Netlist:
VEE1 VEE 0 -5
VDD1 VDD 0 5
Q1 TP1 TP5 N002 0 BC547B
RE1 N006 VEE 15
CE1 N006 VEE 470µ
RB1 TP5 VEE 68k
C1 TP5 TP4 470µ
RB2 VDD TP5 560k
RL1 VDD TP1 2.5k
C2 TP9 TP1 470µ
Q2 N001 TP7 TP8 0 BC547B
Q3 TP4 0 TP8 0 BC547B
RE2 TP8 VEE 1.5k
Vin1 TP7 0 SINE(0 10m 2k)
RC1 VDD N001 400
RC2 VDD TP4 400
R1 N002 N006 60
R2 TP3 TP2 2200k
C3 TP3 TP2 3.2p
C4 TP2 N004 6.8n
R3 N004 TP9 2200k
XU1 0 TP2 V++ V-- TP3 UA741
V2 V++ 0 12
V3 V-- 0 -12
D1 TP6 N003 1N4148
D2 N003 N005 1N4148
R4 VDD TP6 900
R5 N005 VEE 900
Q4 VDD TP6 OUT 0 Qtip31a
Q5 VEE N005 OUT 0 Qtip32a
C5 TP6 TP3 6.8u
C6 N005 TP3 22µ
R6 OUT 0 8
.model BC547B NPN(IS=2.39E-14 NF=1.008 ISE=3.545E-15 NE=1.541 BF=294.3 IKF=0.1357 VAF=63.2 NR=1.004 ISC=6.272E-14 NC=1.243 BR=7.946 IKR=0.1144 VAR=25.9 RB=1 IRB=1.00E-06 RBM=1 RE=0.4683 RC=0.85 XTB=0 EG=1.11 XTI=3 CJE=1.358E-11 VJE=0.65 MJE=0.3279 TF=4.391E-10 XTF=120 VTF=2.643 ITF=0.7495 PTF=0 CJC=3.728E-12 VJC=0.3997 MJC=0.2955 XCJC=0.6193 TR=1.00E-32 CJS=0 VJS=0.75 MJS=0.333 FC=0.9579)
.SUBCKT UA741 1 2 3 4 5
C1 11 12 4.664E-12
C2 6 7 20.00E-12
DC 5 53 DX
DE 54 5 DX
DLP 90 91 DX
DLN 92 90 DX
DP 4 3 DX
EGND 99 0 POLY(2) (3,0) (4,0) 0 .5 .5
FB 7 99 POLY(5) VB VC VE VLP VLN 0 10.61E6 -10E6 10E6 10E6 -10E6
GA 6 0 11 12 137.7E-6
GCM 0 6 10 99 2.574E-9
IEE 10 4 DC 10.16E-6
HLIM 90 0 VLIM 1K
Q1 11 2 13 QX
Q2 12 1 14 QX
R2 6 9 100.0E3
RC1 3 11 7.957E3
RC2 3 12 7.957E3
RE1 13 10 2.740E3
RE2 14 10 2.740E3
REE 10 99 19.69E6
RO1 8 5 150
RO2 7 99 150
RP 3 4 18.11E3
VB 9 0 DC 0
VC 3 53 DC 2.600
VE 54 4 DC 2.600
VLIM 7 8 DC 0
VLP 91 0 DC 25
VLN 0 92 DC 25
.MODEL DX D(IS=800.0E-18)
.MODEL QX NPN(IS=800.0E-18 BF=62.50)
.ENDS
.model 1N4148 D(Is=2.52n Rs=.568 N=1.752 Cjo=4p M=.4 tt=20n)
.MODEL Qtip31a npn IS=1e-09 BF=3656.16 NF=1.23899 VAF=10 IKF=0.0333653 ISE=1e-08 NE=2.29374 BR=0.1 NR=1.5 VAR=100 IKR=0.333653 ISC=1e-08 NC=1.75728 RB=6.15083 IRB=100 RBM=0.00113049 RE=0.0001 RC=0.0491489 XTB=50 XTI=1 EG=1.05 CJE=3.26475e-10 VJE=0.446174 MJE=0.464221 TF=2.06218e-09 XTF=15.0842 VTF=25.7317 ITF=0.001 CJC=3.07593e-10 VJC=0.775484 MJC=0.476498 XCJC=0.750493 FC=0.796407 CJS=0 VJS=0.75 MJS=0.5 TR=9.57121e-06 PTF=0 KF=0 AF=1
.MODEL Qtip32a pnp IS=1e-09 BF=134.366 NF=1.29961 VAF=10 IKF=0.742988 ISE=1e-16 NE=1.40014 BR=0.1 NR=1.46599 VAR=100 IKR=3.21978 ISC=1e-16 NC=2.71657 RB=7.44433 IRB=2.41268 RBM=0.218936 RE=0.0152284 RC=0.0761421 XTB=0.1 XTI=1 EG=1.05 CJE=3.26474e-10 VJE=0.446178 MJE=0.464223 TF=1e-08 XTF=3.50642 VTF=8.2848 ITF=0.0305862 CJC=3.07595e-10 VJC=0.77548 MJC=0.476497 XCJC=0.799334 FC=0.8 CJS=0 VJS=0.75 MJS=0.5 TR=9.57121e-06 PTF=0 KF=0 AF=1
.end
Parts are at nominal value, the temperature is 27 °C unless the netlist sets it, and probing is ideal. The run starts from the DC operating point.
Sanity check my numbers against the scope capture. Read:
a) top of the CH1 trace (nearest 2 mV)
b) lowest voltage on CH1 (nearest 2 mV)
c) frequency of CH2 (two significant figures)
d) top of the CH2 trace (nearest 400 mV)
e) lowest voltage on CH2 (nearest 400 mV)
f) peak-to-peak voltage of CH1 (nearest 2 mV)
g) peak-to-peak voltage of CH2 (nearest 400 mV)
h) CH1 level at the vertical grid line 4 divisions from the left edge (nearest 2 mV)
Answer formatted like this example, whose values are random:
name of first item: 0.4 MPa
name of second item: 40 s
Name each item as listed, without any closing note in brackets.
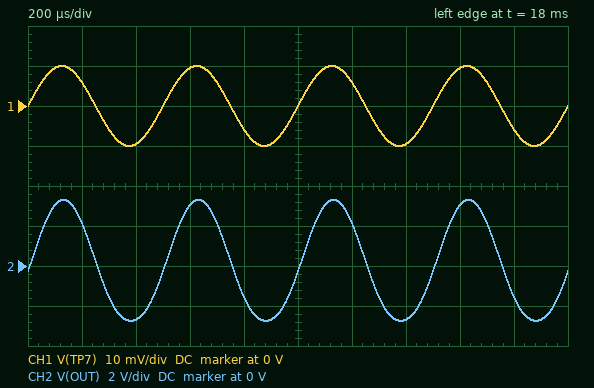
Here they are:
top of the CH1 trace: 10 mV
lowest voltage on CH1: -10 mV
frequency of CH2: 2.0 kHz
top of the CH2 trace: 3.2 V
lowest voltage on CH2: -2.8 V
peak-to-peak voltage of CH1: 20 mV
peak-to-peak voltage of CH2: 6.0 V
CH1 level at the vertical grid line 4 divisions from the left edge: -6 mV
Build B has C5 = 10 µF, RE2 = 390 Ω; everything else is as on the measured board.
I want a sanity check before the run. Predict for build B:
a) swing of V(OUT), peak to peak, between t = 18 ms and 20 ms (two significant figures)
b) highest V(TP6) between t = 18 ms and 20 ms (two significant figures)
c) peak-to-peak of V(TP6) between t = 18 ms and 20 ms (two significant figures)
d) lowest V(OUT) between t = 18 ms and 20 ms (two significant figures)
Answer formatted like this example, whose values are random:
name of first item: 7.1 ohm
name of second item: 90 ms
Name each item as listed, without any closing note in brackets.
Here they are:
swing of V(OUT), peak to peak, between t = 18 ms and 20 ms: 9.4 V
highest V(TP6) between t = 18 ms and 20 ms: 5.6 V
peak-to-peak of V(TP6) between t = 18 ms and 20 ms: 9.8 V
lowest V(OUT) between t = 18 ms and 20 ms: -4.6 V
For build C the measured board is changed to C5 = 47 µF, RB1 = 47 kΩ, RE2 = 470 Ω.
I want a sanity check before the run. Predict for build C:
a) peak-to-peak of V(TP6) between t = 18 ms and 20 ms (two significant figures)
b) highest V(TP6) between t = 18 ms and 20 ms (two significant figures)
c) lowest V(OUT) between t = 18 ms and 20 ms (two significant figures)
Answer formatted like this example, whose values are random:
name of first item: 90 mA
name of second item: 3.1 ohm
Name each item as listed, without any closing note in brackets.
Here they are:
peak-to-peak of V(TP6) between t = 18 ms and 20 ms: 8.8 V
highest V(TP6) between t = 18 ms and 20 ms: 5.6 V
lowest V(OUT) between t = 18 ms and 20 ms: -3.7 V
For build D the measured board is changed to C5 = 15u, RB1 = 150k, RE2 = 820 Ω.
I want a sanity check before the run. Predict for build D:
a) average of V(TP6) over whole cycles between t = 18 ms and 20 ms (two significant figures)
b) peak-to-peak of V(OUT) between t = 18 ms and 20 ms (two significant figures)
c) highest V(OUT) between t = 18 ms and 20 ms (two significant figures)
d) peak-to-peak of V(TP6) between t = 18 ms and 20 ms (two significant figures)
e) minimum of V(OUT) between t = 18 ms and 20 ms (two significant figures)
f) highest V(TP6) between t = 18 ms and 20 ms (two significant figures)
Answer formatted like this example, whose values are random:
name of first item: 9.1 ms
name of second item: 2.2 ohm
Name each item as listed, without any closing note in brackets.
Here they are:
average of V(TP6) over whole cycles between t = 18 ms and 20 ms: 990 mV
peak-to-peak of V(OUT) between t = 18 ms and 20 ms: 7.7 V
highest V(OUT) between t = 18 ms and 20 ms: 3.4 V
peak-to-peak of V(TP6) between t = 18 ms and 20 ms: 7.9 V
minimum of V(OUT) between t = 18 ms and 20 ms: -4.3 V
highest V(TP6) between t = 18 ms and 20 ms: 4.1 V
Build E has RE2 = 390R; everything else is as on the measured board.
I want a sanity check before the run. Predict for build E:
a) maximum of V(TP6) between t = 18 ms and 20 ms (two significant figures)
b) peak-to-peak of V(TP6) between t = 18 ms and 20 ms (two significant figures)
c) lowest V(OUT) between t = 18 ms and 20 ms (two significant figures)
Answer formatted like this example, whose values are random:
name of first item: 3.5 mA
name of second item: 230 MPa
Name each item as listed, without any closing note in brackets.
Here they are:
maximum of V(TP6) between t = 18 ms and 20 ms: 5.6 V
peak-to-peak of V(TP6) between t = 18 ms and 20 ms: 9.8 V
lowest V(OUT) between t = 18 ms and 20 ms: -4.6 V
